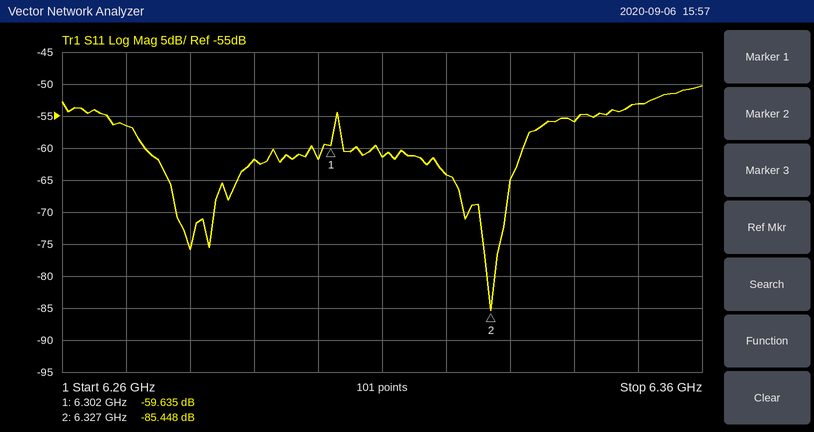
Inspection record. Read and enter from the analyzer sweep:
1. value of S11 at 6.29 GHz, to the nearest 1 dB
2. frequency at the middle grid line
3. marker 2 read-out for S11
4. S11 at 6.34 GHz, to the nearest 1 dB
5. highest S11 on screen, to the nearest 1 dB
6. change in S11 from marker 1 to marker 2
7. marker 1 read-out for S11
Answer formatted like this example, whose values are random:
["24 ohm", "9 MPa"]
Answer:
["-62 dB", "6.31 GHz", "-85.448 dB", "-56 dB", "-50 dB", "-25.813 dB", "-59.635 dB"]
